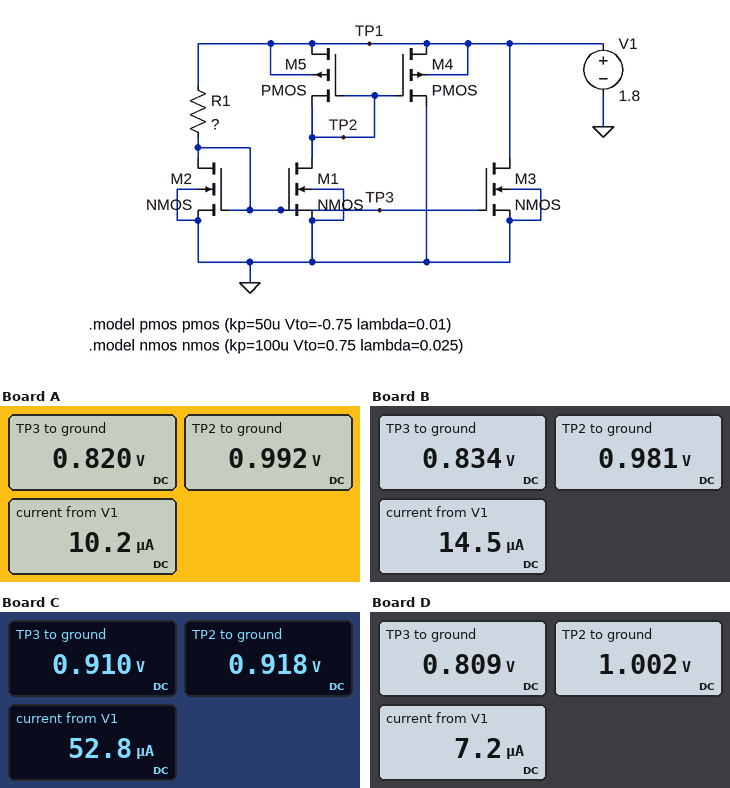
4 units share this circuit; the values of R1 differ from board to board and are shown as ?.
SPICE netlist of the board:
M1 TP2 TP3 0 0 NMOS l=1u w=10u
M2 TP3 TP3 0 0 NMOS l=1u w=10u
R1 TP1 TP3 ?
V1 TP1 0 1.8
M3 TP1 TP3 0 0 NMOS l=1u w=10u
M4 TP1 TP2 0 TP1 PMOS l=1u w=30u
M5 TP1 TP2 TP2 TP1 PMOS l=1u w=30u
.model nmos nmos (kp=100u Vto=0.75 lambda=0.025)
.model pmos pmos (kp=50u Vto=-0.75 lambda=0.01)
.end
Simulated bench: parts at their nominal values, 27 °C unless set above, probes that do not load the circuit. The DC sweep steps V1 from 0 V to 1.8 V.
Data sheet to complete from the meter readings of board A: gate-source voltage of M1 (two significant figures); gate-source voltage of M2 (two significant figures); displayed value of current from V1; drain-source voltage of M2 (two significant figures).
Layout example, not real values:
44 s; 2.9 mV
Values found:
820 mV; 820 mV; 10.2 µA; 820 mV
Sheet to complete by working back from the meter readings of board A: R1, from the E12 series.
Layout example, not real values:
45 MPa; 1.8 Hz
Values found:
390 kΩ
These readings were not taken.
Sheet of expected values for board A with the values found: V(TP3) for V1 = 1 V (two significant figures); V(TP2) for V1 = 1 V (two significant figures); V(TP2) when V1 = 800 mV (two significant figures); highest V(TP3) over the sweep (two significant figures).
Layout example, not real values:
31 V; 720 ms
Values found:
780 mV; 220 mV; 39 mV; 820 mV
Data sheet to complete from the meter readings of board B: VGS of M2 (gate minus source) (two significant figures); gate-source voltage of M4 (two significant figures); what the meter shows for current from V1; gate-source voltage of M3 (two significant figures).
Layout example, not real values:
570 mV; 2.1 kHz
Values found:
830 mV; 980 mV; 14.5 µA; 830 mV
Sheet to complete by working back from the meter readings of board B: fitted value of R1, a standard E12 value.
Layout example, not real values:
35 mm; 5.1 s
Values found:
270 kΩ
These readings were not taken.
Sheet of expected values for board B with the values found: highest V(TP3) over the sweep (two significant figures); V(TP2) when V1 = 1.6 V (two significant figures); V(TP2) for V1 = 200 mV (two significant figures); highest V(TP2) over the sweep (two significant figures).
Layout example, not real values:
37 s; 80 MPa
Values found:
830 mV; 790 mV; 100 mV; 980 mV
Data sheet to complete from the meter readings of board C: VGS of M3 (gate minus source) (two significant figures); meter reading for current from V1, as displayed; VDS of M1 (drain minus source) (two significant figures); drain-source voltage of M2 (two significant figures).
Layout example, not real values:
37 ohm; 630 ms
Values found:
910 mV; 52.8 µA; 920 mV; 910 mV
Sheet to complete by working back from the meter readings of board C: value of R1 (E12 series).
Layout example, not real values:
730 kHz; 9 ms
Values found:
68 kΩ
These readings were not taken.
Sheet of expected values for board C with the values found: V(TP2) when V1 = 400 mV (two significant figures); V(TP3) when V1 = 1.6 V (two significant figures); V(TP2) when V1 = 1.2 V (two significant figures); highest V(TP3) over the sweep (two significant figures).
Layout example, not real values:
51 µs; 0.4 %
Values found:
200 mV; 890 mV; 370 mV; 910 mV
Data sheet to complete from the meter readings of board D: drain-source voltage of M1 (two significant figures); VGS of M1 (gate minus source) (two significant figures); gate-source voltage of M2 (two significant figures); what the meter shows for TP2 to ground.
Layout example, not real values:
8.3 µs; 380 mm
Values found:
1.0 V; 810 mV; 810 mV; 1.002 V
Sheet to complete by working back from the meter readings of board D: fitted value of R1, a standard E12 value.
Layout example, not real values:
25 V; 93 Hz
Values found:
560 kΩ
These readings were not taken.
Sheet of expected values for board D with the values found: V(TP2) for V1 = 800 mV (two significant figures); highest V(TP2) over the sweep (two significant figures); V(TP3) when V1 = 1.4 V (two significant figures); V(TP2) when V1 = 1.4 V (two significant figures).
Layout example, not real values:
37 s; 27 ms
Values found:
41 mV; 1.0 V; 800 mV; 610 mV
